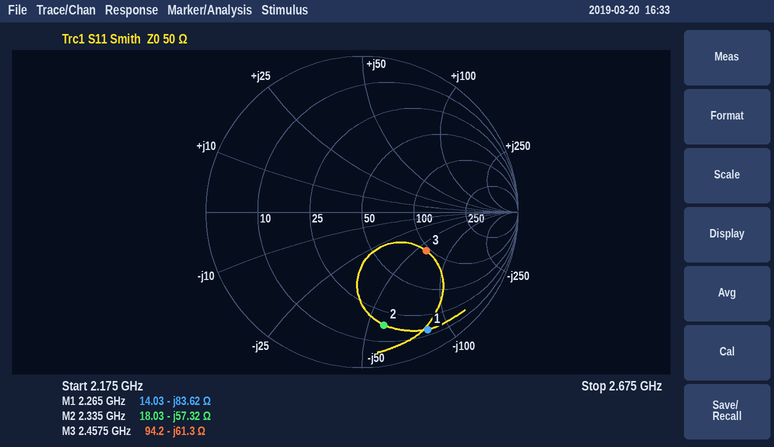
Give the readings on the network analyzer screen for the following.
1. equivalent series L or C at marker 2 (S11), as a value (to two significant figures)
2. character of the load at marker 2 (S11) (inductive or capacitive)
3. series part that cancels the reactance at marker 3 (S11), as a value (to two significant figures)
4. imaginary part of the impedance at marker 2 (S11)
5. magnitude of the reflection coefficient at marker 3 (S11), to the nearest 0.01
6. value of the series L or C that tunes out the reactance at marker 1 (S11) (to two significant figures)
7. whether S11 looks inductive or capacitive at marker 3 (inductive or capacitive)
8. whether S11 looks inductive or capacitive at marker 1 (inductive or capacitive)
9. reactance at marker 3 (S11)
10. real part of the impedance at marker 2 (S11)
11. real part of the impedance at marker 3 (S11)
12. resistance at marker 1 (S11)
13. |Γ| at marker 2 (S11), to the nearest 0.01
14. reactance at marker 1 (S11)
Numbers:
1.2 pF
capacitive
4.0 nH
-57.32 Ω
0.48
5.9 nH
capacitive
capacitive
-61.3 Ω
18.03 Ω
94.2 Ω
14.03 Ω
0.74
-83.62 Ω
